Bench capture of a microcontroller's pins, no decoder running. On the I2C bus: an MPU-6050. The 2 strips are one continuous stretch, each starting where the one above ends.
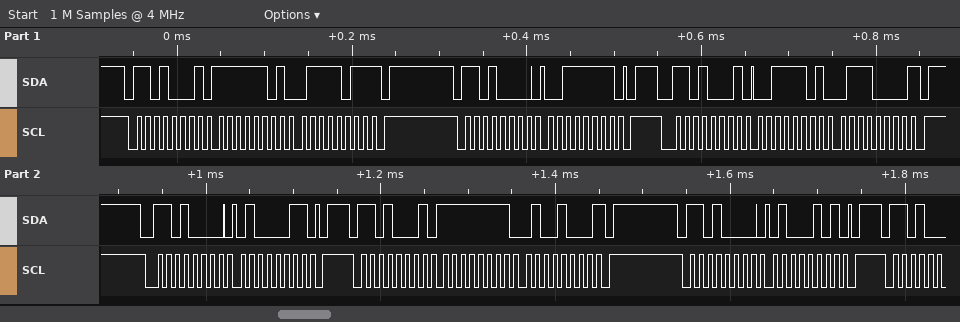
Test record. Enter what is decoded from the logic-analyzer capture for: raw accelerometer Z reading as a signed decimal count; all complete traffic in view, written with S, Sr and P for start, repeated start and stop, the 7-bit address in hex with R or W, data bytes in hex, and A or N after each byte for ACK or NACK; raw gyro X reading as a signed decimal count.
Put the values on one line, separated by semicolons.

15728; S 68R A FD A 7B N P S 68W A 3F A P S 68R A 3D A 70 N P S 68W A 43 A P S 68R A FF A 48 N P S 68W A 45 A P; -184
